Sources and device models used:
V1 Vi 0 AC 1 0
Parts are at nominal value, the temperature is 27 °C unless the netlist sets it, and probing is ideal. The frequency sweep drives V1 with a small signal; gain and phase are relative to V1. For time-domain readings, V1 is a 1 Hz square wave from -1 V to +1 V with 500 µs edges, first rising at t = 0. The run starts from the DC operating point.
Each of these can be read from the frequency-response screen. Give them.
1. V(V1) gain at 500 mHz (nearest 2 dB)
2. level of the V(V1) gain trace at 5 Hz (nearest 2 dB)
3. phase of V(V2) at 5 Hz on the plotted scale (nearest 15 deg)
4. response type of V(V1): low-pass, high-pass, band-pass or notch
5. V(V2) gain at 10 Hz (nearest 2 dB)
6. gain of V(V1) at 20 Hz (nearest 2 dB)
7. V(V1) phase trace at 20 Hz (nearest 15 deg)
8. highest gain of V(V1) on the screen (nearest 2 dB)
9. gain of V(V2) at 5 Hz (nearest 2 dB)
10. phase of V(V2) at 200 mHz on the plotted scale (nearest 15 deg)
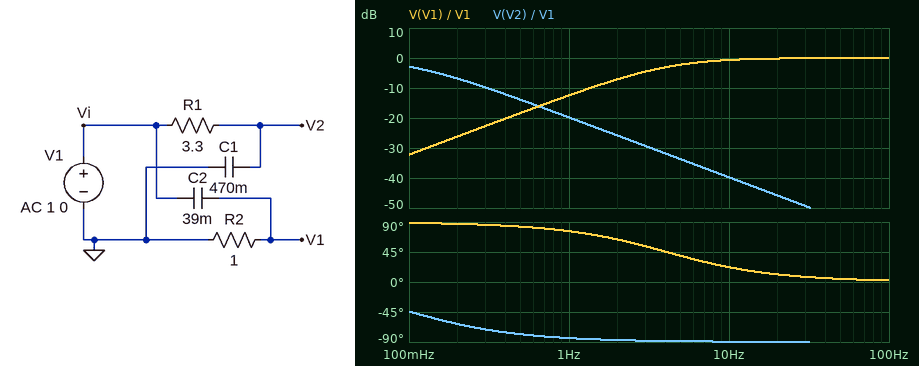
-18 dB
-2 dB
-90 deg
high-pass
-40 dB
0 dB
15 deg
0 dB
-34 dB
-60 deg
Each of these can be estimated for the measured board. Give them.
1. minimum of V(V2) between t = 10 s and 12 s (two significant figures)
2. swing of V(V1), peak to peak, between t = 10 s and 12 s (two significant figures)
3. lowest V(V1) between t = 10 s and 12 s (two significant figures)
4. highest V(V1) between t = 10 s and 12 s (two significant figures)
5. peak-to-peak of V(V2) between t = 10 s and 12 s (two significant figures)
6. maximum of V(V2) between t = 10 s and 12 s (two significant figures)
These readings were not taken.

-160 mV
4.0 V
-2.0 V
2.0 V
320 mV
160 mV
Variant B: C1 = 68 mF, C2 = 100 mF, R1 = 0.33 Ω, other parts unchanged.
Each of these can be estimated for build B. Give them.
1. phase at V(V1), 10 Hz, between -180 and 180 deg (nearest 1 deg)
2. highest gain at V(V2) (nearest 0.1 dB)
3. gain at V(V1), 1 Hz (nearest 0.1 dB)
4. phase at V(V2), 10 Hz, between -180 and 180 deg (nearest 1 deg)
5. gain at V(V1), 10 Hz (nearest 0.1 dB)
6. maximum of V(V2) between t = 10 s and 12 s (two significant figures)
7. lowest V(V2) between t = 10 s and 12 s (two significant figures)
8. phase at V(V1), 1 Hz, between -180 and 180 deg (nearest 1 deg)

9 deg
0 dB
-5.5 dB
-55 deg
-0.1 dB
1.0 V
-1.0 V
58 deg
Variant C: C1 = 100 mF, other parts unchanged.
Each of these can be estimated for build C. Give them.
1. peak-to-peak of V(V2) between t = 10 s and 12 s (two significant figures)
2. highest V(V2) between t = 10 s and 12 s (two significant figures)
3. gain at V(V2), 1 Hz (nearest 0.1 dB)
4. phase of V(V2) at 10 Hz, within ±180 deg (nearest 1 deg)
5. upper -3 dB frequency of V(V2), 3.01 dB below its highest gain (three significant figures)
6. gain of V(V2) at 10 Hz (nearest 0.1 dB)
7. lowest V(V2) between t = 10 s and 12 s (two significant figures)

1.3 V
640 mV
-7.2 dB
-87 deg
482 mHz
-26.3 dB
-640 mV
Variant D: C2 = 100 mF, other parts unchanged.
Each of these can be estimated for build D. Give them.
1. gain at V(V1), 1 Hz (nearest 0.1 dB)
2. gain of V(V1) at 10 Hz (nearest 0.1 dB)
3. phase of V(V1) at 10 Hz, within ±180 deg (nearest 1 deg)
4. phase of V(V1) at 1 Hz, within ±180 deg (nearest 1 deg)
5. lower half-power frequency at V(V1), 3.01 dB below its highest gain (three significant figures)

-5.5 dB
-0.1 dB
9 deg
58 deg
1.59 Hz
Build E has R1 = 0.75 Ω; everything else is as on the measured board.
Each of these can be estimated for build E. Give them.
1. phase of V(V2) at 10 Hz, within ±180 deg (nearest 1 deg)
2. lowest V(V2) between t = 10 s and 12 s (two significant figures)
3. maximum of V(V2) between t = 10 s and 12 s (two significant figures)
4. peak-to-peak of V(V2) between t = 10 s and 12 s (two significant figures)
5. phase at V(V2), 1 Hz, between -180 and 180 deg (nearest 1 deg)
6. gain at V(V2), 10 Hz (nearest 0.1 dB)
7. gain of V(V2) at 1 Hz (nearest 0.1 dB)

-87 deg
-610 mV
610 mV
1.2 V
-66 deg
-26.9 dB
-7.7 dB
